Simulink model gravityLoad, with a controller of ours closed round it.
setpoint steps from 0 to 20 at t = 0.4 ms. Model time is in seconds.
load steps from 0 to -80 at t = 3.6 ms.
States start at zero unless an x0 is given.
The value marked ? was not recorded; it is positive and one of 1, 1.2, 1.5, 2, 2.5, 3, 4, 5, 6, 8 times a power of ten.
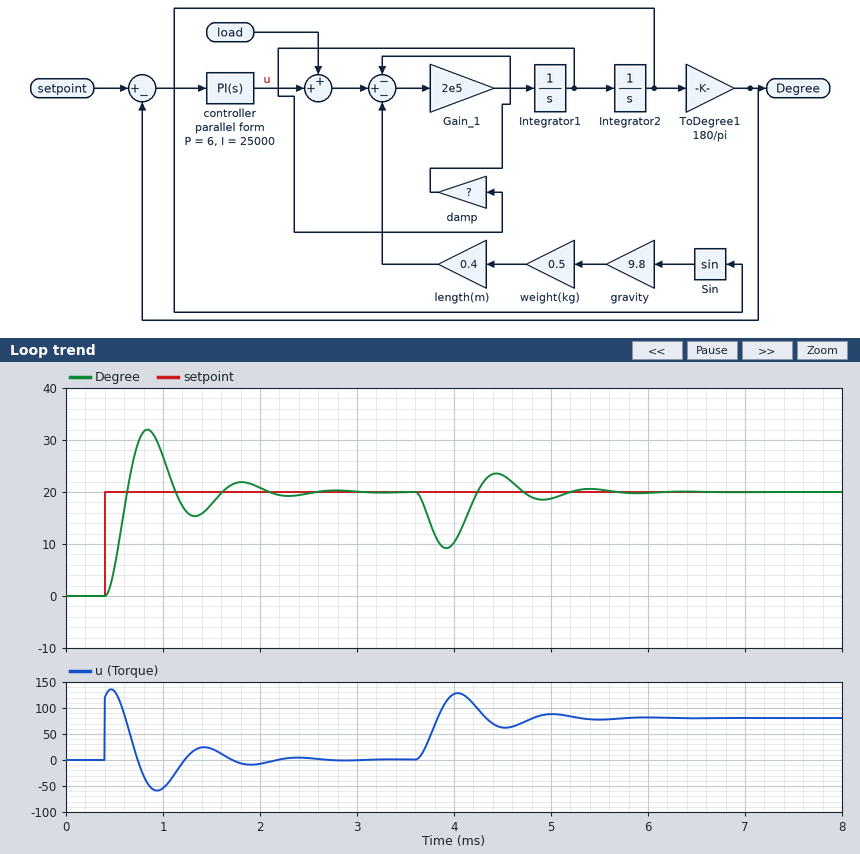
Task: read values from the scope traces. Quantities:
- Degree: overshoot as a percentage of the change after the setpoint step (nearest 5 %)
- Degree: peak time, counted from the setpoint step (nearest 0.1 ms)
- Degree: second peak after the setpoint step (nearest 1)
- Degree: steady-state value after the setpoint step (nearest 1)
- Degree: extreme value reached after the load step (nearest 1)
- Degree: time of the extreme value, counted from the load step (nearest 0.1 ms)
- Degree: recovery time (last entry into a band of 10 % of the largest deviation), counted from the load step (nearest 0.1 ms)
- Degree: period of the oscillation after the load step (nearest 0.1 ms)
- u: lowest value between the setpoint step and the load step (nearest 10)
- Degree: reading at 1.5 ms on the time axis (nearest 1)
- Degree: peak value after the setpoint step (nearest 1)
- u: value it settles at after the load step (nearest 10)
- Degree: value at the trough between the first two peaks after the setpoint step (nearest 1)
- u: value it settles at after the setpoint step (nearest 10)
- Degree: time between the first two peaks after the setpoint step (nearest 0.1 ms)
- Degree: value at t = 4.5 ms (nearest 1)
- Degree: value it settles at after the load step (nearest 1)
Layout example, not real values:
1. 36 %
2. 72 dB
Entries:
1. 60 %
2. 0.4 ms
3. 22
4. 20
5. 9
6. 0.3 ms
7. 1.4 ms
8. 1.0 ms
9. -60
10. 18
11. 32
12. 80
13. 15
14. 0
15. 1.0 ms
16. 23
17. 20
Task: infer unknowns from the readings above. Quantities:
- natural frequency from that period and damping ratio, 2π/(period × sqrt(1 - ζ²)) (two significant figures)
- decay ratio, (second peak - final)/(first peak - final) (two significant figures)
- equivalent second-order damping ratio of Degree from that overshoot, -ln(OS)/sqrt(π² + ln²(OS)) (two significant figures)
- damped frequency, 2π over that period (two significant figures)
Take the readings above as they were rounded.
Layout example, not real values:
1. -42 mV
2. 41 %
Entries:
1. 6.4 rad/ms
2. 0.17
3. 0.16
4. 6.3 rad/ms
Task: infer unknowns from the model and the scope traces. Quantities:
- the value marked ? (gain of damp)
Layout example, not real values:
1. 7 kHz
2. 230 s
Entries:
1. 0.05
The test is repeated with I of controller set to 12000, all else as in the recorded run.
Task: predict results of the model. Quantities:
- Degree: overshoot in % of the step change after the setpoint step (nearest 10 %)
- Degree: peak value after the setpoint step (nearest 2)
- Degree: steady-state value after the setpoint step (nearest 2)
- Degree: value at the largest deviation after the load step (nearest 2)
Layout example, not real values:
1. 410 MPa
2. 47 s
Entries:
1. 40 %
2. 28
3. 20
4. 8
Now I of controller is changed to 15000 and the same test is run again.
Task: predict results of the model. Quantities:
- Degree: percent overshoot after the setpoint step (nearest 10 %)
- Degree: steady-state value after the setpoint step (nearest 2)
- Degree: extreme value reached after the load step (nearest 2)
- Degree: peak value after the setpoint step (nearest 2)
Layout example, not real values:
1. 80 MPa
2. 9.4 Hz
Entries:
1. 40 %
2. 20
3. 8
4. 28
